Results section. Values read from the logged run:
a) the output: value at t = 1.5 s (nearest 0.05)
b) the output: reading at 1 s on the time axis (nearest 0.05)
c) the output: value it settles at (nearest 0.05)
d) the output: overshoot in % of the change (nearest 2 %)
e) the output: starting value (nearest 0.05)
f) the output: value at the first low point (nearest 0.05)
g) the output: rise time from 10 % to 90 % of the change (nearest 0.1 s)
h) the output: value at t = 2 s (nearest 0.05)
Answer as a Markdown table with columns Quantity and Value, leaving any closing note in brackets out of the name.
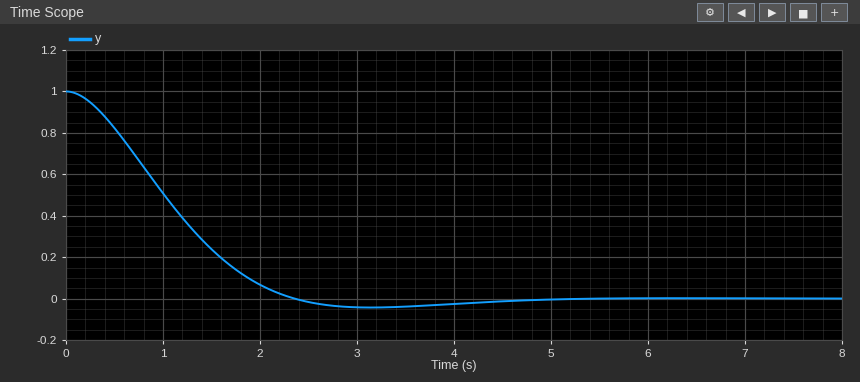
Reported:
| Quantity | Value |
|---|---|
| the output: value at t = 1.5 s | 0.25 |
| the output: reading at 1 s on the time axis | 0.50 |
| the output: value it settles at | 0.00 |
| the output: overshoot in % of the change | 4 % |
| the output: starting value | 1.00 |
| the output: value at the first low point | -0.05 |
| the output: rise time from 10 % to 90 % of the change | 1.5 s |
| the output: value at t = 2 s | 0.05 |
